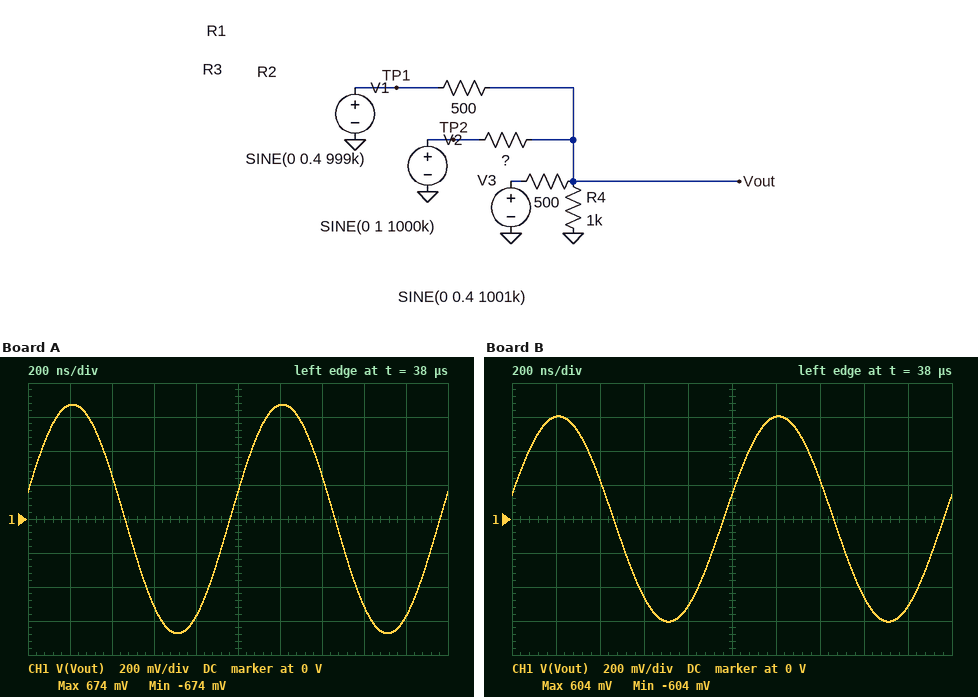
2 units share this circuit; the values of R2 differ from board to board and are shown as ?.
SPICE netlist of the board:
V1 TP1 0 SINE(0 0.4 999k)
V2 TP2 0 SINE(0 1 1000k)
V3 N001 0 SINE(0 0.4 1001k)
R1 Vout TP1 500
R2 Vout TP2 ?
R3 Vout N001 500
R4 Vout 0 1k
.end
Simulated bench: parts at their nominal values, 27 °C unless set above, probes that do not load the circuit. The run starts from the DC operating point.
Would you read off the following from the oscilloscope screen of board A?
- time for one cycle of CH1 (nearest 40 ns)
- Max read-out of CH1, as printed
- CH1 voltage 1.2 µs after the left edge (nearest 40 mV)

1.00 µs
674 mV
680 mV
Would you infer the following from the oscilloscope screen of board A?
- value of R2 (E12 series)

180 Ω
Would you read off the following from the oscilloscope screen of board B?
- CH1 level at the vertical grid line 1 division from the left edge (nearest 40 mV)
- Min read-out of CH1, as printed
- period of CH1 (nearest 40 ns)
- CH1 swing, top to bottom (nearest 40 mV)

600 mV
-604 mV
1.00 µs
1.20 V
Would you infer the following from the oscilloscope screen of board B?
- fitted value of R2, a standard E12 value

270 Ω
